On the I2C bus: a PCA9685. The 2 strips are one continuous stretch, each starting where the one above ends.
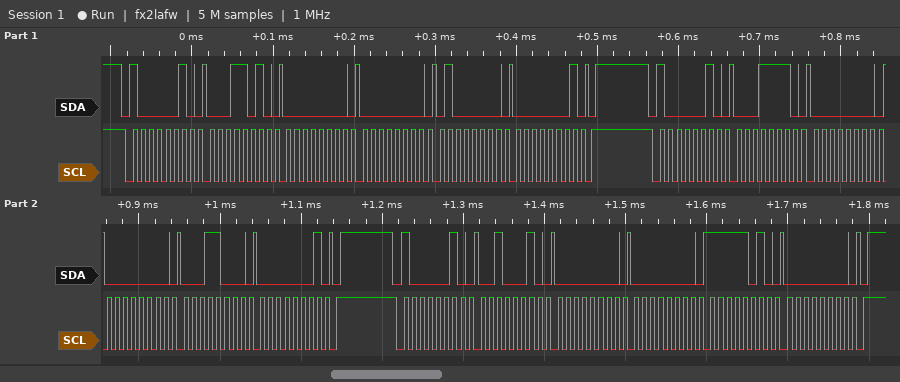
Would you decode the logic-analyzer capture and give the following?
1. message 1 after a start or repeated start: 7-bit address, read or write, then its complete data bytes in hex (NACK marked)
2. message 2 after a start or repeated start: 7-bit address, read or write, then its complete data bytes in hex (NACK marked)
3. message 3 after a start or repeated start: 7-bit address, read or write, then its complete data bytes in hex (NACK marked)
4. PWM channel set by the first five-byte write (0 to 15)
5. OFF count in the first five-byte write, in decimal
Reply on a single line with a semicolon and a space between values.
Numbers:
0x41 write: 1A 00 00 40 01; 0x41 write: 1E 00 00 18 01; 0x41 write: 22 00 00 FA 00; 5; 320
